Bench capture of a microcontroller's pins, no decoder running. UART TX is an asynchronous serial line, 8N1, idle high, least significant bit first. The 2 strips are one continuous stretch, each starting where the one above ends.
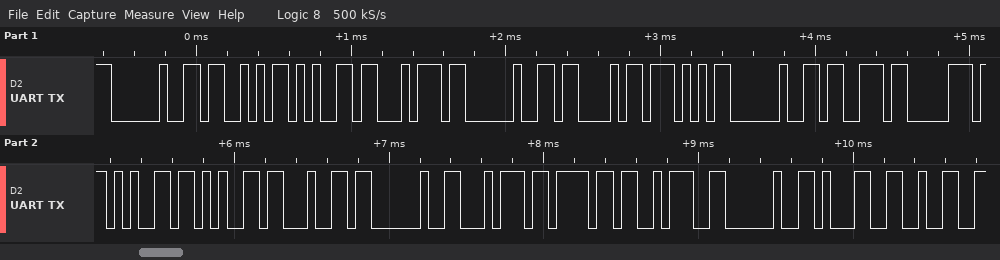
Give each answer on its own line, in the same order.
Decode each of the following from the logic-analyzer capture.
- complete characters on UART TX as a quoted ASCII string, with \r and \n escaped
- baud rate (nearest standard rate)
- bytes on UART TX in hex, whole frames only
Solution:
" Set CW speed to: 12"
19200 baud
0x20 0x53 0x65 0x74 0x20 0x43 0x57 0x20 0x73 0x70 0x65 0x65 0x64 0x20 0x74 0x6F 0x3A 0x20 0x31 0x32
